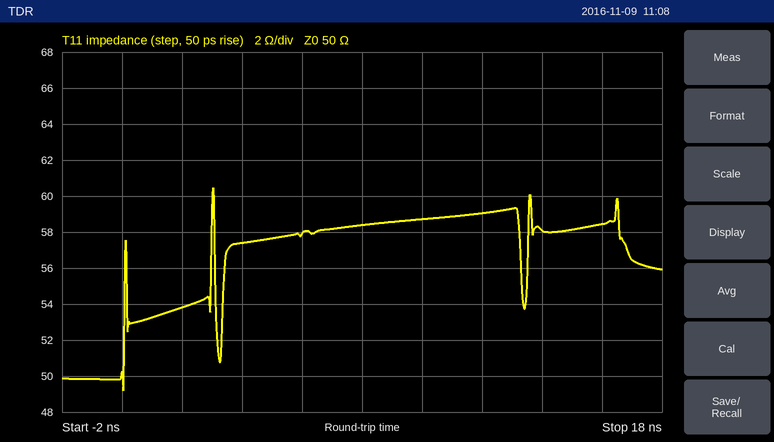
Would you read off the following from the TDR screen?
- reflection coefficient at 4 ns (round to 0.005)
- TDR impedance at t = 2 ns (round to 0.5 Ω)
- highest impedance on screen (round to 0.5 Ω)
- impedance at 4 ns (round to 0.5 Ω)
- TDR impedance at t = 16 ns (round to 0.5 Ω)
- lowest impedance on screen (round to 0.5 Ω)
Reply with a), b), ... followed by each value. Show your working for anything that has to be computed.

a) (57.5 − 50)/(57.5 + 50) ≈ +0.070
b) 54.0 Ω
c) 60.5 Ω
d) 57.5 Ω
e) 58.5 Ω
f) 49.0 Ω
